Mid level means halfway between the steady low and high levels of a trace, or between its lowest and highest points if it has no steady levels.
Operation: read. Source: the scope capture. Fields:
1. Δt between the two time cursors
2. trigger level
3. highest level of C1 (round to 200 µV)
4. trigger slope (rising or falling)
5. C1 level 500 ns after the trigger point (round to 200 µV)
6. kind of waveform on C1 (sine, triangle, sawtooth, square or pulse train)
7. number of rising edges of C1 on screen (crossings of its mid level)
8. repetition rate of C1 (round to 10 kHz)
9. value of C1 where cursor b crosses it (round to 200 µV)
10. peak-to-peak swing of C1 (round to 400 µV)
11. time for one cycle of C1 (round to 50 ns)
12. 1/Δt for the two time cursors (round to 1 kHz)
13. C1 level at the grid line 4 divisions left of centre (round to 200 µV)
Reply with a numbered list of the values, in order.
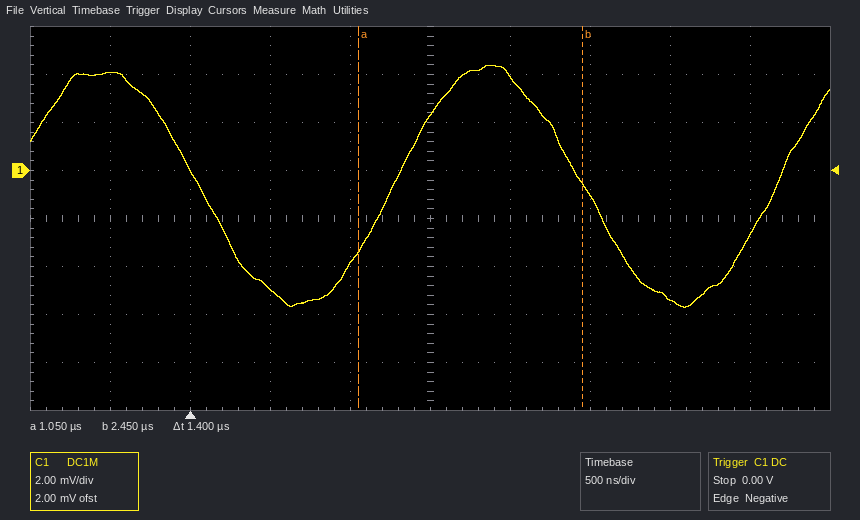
1. 1.4 µs
2. 0.00 V
3. 4.4 mV
4. falling
5. -5.0 mV
6. sine
7. 2
8. 420 kHz
9. -600 µV
10. 10.0 mV
11. 2.40 µs
12. 714 kHz
13. 4.0 mV
